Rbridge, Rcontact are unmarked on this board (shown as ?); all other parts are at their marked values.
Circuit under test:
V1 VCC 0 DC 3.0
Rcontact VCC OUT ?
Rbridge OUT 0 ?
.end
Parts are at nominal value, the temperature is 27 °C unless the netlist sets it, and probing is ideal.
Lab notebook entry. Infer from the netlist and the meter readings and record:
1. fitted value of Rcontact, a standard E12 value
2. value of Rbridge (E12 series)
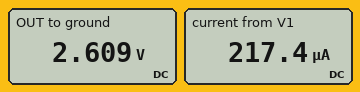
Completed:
1.8 kΩ
12 kΩ
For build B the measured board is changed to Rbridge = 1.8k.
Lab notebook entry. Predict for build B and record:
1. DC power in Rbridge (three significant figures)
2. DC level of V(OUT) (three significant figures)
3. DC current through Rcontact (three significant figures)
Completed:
1.25 mW
1.50 V
833 µA
